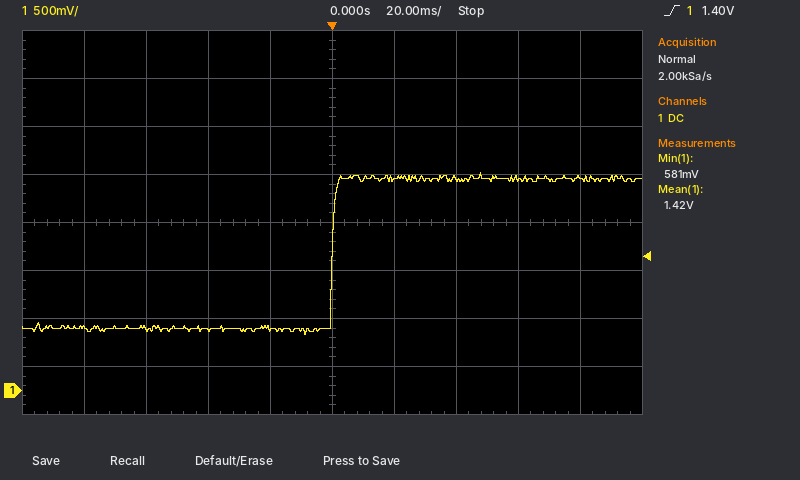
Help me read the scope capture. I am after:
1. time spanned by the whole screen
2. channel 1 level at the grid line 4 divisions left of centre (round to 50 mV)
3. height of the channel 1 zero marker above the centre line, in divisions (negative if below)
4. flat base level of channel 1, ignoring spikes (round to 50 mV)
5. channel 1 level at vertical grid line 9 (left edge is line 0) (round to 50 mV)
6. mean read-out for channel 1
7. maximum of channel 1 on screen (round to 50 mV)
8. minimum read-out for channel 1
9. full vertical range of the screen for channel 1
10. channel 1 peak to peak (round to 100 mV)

200 ms
650 mV
-3.5 div
650 mV
2.20 V
1.42 V
2.25 V
581 mV
4 V
1.70 V
